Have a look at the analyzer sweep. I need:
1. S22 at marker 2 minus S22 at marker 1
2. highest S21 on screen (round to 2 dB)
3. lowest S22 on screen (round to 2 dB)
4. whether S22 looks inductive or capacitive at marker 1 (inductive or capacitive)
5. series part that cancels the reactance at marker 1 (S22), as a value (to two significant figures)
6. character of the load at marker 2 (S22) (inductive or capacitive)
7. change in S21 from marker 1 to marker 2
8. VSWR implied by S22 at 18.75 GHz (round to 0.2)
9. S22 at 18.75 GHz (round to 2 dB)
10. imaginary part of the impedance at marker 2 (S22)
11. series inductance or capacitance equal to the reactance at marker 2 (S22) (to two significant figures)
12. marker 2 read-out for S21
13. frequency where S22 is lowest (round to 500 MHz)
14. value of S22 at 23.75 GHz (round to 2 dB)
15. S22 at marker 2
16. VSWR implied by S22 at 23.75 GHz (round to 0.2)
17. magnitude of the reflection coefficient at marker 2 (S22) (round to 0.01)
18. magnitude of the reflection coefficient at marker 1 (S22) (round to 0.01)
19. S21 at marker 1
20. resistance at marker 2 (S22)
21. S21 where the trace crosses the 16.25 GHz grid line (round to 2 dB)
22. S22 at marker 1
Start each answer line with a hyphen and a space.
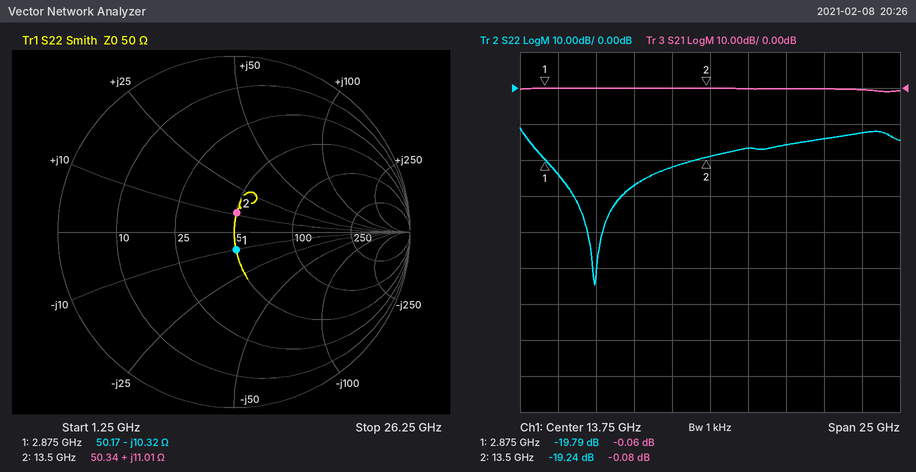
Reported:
- 0.55 dB
- 0 dB
- -54 dB
- capacitive
- 570 pH
- inductive
- -0.02 dB
- 1.4
- -16 dB
- +11.01 Ω
- 130 pH
- -0.08 dB
- 6.0 GHz
- -12 dB
- -19.24 dB
- 1.6
- 0.11
- 0.10
- -0.06 dB
- 50.34 Ω
- 0 dB
- -19.79 dB
